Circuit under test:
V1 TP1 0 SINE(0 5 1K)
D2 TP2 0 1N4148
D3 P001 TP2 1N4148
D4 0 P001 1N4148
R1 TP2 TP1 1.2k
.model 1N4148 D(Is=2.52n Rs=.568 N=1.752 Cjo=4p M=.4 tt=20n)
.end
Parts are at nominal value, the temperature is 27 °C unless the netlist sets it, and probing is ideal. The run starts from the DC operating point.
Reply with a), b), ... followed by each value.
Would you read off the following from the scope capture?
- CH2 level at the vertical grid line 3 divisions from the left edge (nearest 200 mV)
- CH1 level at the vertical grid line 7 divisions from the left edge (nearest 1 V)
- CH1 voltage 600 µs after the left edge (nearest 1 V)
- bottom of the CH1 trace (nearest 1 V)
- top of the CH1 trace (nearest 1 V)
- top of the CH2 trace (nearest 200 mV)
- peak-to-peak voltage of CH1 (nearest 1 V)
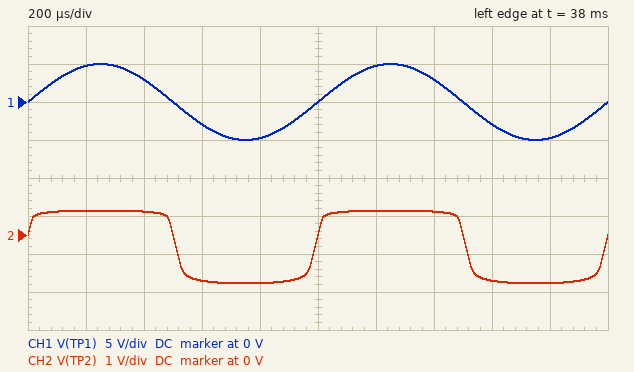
a) -1.2 V
b) 3 V
c) -3 V
d) -5 V
e) 5 V
f) 600 mV
g) 10 V
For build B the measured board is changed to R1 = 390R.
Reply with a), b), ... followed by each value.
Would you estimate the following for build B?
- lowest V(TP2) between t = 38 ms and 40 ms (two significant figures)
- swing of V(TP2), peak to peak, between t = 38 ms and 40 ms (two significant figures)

a) -1.4 V
b) 2.1 V
